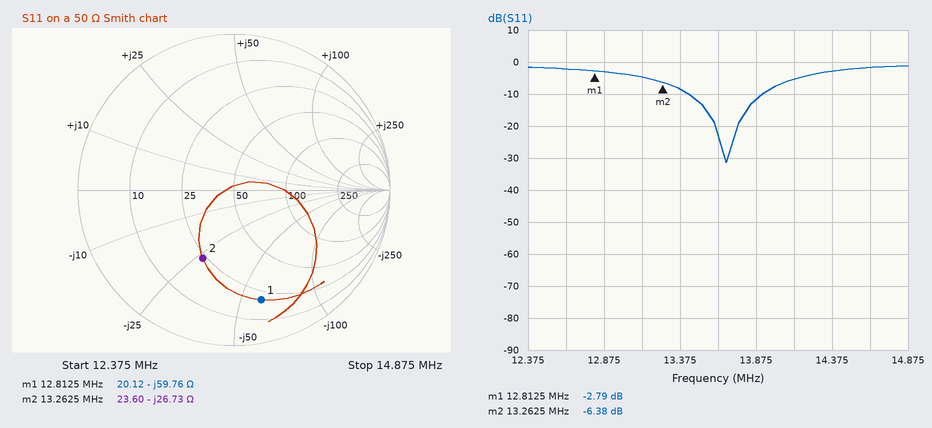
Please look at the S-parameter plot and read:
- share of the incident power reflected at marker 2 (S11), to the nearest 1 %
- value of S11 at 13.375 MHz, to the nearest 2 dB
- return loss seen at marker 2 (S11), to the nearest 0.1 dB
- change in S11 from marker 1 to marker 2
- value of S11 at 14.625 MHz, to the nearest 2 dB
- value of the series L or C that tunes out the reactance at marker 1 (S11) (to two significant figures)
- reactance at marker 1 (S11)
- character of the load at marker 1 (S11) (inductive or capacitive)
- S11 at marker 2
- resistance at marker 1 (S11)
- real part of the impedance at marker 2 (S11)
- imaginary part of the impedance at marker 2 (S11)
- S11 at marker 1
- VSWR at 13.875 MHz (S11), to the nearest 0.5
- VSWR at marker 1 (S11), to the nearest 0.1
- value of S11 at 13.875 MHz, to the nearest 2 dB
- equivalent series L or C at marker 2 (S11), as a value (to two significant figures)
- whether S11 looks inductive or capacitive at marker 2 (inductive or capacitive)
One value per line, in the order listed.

23 %
-8 dB
6.4 dB
-3.59 dB
-2 dB
740 nH
-59.76 Ω
capacitive
-6.38 dB
20.12 Ω
23.60 Ω
-26.73 Ω
-2.79 dB
1.5
6.3
-12 dB
450 pF
capacitive
